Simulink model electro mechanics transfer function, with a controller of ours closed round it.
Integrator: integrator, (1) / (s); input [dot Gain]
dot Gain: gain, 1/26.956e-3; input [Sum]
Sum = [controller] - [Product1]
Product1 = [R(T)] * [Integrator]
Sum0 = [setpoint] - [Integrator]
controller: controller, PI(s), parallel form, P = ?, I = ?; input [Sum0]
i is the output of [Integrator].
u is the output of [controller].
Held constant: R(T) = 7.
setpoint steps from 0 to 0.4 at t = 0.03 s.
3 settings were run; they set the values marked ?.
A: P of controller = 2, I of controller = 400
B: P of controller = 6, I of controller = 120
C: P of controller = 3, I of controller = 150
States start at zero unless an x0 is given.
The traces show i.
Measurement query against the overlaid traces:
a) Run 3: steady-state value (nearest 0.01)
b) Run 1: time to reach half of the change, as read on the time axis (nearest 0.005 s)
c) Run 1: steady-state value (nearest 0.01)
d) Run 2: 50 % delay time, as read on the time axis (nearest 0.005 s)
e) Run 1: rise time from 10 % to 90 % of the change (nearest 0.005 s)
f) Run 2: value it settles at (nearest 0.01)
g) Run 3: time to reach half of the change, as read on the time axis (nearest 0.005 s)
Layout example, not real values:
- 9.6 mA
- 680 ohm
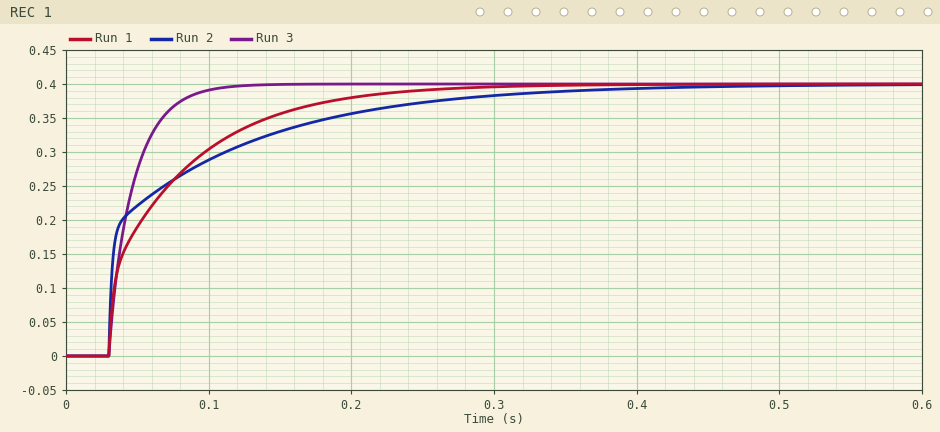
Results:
- 0.40
- 0.055 s
- 0.40
- 0.040 s
- 0.125 s
- 0.40
- 0.040 s
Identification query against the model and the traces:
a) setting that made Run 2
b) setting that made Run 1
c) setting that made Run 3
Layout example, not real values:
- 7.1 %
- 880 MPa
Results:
- B
- C
- A
